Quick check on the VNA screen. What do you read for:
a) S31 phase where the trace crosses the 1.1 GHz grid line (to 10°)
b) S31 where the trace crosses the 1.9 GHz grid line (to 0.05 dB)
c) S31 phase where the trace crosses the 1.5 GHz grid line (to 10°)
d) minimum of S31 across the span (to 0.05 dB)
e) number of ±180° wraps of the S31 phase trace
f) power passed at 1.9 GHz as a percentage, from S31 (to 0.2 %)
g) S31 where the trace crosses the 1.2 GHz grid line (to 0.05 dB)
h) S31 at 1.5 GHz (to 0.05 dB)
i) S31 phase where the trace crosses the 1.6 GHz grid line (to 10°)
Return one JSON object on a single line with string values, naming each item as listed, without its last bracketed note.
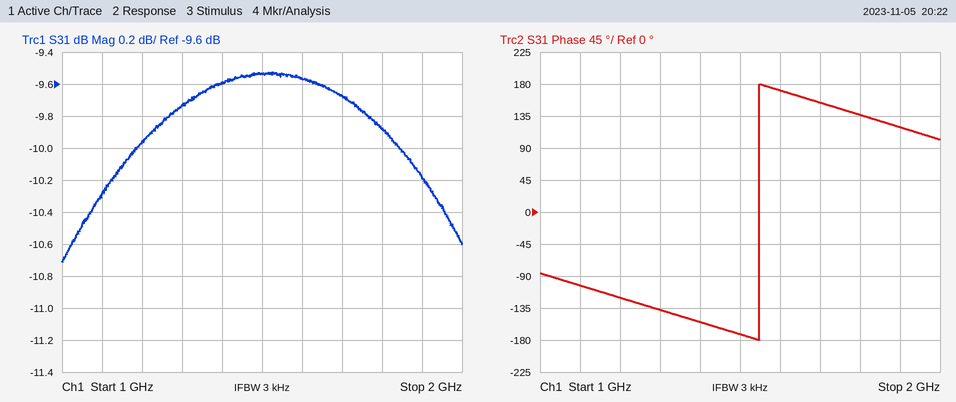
{"S31 phase where the trace crosses the 1.1 GHz grid line": "-100°", "S31 where the trace crosses the 1.9 GHz grid line": "-10.20 dB", "S31 phase where the trace crosses the 1.5 GHz grid line": "-170°", "minimum of S31 across the span": "-10.70 dB", "number of ±180° wraps of the S31 phase trace": "1", "power passed at 1.9 GHz as a percentage, from S31": "9.6 %", "S31 where the trace crosses the 1.2 GHz grid line": "-9.95 dB", "S31 at 1.5 GHz": "-9.55 dB", "S31 phase where the trace crosses the 1.6 GHz grid line": "170°"}
